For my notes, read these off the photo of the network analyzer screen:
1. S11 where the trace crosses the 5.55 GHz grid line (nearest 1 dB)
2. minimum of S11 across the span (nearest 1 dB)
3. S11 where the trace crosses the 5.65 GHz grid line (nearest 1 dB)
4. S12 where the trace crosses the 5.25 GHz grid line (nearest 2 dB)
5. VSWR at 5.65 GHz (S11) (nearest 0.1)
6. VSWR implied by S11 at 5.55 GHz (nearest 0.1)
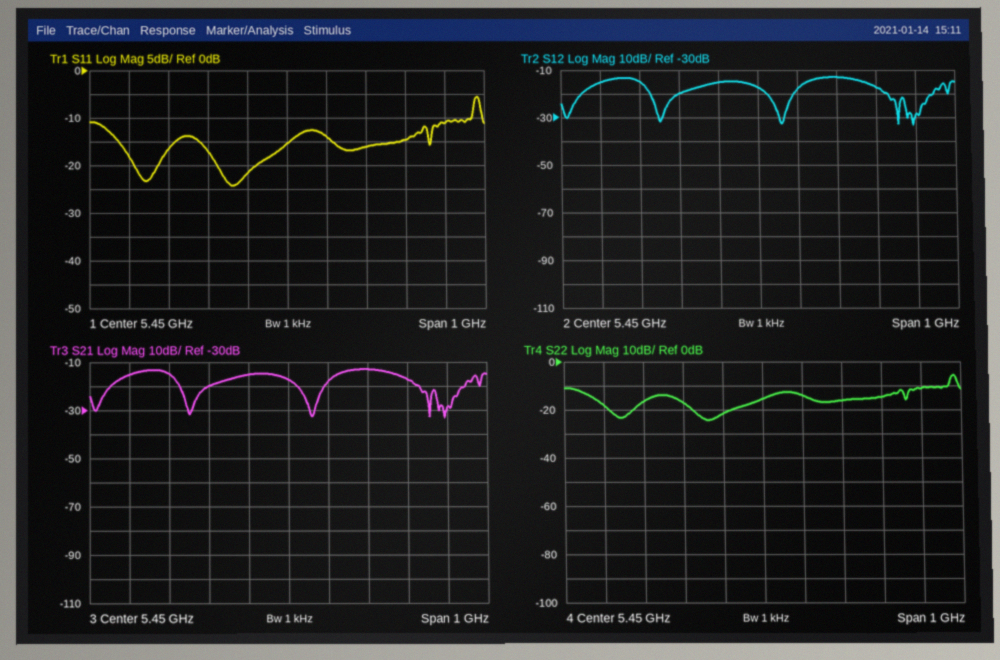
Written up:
-14 dB
-24 dB
-16 dB
-20 dB
1.4
1.5
